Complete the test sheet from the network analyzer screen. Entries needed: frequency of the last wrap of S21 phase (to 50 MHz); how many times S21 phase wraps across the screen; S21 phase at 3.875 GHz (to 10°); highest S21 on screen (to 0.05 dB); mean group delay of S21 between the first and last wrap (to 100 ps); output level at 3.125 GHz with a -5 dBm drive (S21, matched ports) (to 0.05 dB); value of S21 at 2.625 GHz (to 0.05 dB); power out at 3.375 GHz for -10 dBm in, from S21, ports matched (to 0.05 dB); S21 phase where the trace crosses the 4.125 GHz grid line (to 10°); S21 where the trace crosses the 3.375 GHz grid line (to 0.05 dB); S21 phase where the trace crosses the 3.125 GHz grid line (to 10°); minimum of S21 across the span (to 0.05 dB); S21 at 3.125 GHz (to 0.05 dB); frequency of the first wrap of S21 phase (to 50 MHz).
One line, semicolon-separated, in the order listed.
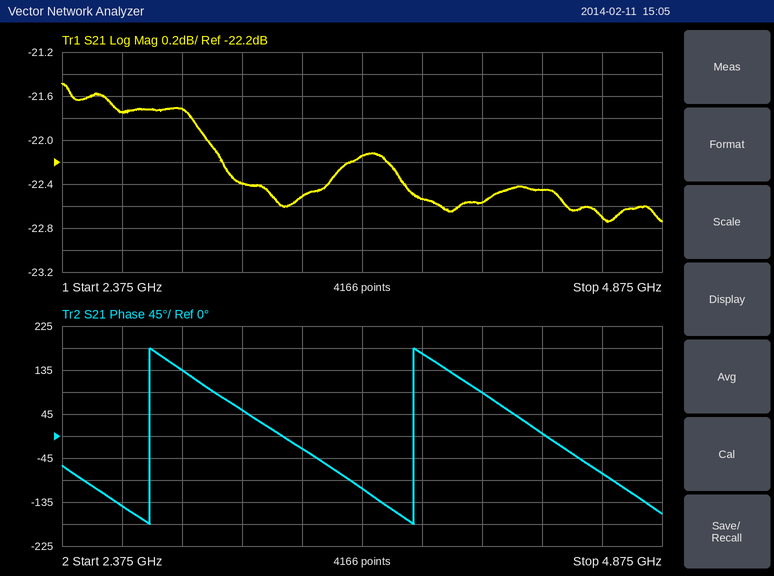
3.85 GHz; 2; 170°; -21.50 dB; 900 ps; -27.40 dBm; -21.75 dB; -32.50 dBm; 90°; -22.50 dB; 50°; -22.75 dB; -22.40 dB; 2.75 GHz
